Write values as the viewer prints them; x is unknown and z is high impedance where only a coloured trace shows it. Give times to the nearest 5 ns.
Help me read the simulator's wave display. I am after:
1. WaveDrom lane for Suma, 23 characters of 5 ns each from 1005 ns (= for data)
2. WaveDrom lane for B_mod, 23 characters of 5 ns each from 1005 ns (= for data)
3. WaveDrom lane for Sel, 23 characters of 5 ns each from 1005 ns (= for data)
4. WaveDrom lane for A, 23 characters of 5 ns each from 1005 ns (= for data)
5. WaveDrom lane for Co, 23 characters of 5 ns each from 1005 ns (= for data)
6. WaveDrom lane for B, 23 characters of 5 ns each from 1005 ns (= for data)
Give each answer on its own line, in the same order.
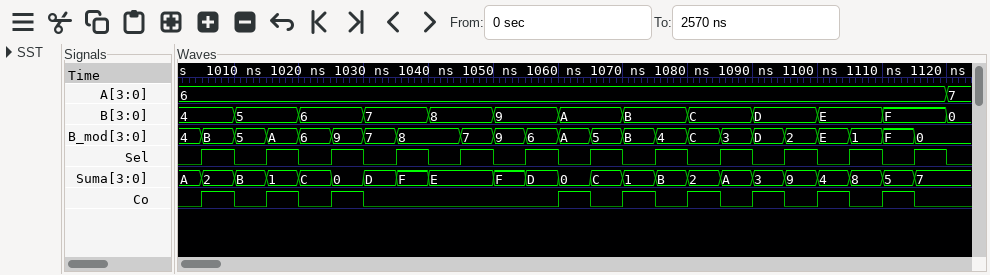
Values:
{name: 'Suma', wave: '========.==============', data: '2 B 1 C 0 D F E F D 0 C 1 B 2 A 3 9 4 8 5 7'}
{name: 'B_mod', wave: '=======.===============', data: 'B 5 A 6 9 7 8 7 9 6 A 5 B 4 C 3 D 2 E 1 F 0'}
{name: 'Sel', wave: '10101010101010101010101'}
{name: 'A', wave: '=......................', data: '6'}
{name: 'Co', wave: '101010.....101010101010'}
{name: 'B', wave: '==.=.=.=.=.=.=.=.=.=.=.', data: '4 5 6 7 8 9 A B C D E F'}
